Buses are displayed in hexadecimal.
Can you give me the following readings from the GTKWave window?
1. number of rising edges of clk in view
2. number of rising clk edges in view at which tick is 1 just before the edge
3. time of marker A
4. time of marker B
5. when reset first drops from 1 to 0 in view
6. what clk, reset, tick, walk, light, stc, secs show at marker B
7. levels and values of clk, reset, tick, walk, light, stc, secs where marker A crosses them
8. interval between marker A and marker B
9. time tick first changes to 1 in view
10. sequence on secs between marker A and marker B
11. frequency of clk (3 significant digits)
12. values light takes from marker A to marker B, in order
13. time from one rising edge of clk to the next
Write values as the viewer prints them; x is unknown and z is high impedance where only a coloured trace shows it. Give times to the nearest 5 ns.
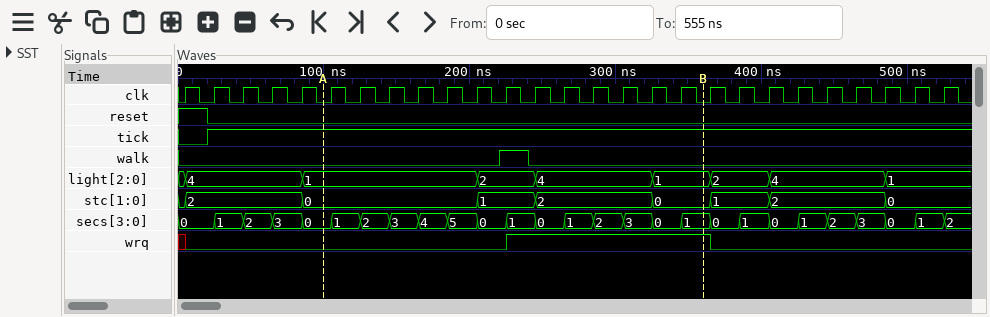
27
26
100 ns
360 ns
20 ns
clk=0, reset=0, tick=1, walk=0, light=1, stc=0, secs=1
clk=0, reset=0, tick=1, walk=0, light=1, stc=0, secs=0
260 ns
20 ns
0, 1, 2, 3, 4, 5, 0, 1, 0, 1, 2, 3, 0, 1
50.0 MHz
1, 2, 4, 1
20 ns
